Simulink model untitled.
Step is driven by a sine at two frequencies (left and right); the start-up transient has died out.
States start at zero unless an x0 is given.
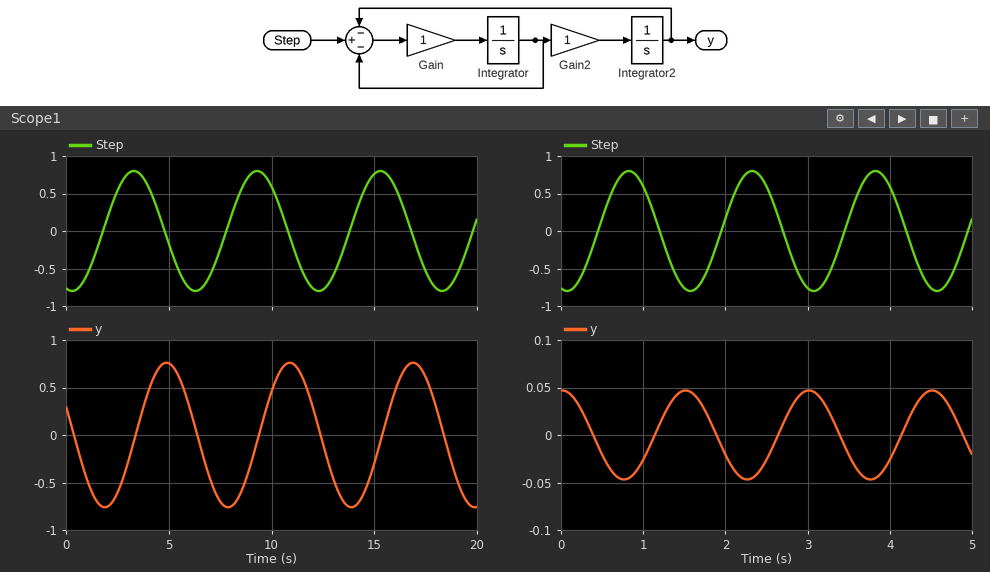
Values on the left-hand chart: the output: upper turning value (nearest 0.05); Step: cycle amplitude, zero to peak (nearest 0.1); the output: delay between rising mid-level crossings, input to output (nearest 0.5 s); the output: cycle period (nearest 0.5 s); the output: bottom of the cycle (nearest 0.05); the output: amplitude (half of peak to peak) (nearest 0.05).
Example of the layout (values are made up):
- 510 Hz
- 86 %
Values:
- 0.75
- 0.8
- 1.5 s
- 6.0 s
- -0.75
- 0.75
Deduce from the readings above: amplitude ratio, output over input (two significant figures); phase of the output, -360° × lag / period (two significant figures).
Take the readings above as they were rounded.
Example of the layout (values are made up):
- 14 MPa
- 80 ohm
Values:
- 0.94
- -90°
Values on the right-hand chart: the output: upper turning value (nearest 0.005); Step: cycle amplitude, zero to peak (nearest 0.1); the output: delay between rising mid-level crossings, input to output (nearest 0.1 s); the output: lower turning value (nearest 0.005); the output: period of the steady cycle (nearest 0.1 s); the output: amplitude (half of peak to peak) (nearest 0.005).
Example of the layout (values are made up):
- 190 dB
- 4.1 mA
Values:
- 0.045
- 0.8
- 0.7 s
- -0.045
- 1.5 s
- 0.045
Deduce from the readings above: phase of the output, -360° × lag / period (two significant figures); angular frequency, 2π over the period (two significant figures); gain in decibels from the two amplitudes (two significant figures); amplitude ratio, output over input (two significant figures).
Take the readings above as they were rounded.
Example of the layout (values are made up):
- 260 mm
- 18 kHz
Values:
- -170°
- 4.2 rad/s
- -25 dB
- 0.056
